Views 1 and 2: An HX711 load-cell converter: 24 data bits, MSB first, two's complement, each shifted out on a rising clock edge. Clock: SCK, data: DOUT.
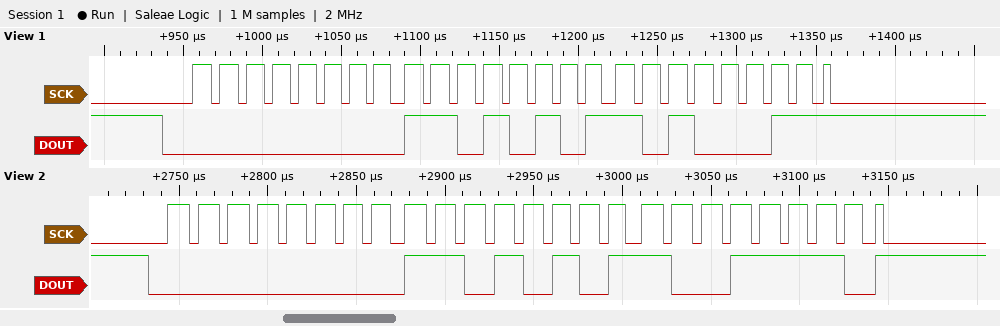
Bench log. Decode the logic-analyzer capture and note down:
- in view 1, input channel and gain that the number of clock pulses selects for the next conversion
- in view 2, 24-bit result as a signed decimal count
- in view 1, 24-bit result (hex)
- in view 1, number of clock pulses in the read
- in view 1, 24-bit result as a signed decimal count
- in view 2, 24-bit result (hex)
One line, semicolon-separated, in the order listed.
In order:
channel A, gain 128; 54686; 0x00D5A3; 25; 54691; 0x00D59E
